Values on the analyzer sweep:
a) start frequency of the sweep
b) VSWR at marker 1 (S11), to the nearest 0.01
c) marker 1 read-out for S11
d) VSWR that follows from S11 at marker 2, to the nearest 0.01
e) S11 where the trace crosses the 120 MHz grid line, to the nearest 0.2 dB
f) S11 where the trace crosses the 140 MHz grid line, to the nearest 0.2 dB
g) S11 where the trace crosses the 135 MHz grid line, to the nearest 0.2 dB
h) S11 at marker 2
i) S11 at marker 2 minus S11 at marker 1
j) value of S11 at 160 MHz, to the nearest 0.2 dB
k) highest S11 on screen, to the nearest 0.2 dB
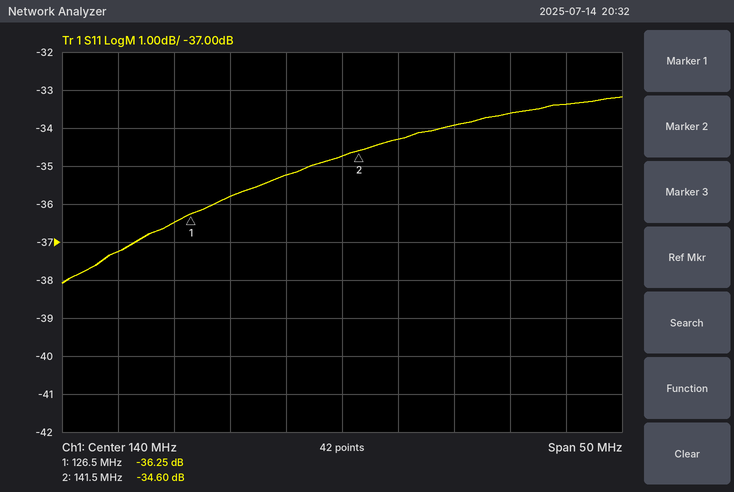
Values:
115 MHz
1.03
-36.25 dB
1.04
-37.2 dB
-34.8 dB
-35.2 dB
-34.60 dB
1.65 dB
-33.4 dB
-33.2 dB
